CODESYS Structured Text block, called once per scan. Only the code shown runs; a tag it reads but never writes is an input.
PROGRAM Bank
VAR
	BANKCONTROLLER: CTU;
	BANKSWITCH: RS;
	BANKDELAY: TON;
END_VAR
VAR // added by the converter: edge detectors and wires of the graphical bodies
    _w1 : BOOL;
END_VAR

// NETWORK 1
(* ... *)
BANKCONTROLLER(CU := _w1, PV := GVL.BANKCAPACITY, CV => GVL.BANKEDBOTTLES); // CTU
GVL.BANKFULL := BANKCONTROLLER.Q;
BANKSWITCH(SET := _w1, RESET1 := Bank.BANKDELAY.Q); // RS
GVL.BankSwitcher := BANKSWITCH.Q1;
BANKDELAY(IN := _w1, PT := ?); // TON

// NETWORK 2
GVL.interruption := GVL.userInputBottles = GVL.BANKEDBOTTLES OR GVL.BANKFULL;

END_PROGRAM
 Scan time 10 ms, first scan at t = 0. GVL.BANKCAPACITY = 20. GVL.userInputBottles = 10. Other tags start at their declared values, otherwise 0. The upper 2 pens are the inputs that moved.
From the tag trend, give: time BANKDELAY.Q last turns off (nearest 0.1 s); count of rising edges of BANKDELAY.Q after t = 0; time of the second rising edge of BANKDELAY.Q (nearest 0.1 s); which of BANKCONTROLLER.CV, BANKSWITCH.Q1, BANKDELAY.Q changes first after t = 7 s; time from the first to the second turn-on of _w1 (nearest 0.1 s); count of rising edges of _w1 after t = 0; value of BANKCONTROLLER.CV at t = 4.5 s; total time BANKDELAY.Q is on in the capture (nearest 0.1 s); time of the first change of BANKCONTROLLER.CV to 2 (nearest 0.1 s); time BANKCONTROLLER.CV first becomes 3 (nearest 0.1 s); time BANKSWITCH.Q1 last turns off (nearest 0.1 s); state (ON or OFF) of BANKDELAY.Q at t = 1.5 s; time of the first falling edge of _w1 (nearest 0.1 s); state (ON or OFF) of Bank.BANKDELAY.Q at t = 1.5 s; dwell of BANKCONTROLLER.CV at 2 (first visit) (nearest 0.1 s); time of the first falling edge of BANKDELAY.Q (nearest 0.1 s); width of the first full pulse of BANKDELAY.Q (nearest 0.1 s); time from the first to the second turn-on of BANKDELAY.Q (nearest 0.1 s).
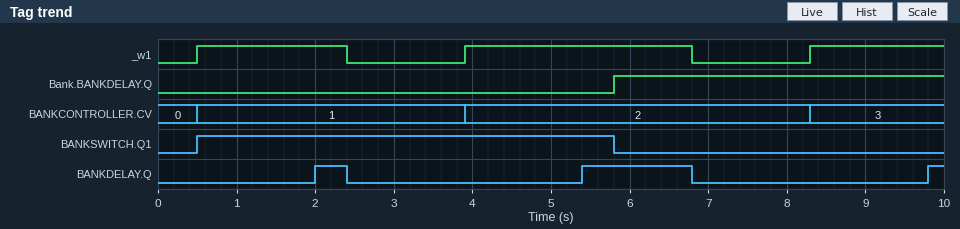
6.8 s
3
5.4 s
BANKCONTROLLER.CV
3.4 s
3
2
2.0 s
3.9 s
8.3 s
5.8 s
OFF
2.4 s
OFF
4.4 s
2.4 s
0.4 s
3.4 s
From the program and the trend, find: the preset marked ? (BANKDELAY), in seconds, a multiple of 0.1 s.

1.5 s
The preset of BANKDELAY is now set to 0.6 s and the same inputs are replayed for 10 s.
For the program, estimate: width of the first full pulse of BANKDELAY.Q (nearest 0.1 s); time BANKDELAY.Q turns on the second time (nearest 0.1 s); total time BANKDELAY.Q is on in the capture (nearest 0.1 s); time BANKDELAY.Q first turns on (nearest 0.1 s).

1.3 s
4.5 s
4.7 s
1.1 s
